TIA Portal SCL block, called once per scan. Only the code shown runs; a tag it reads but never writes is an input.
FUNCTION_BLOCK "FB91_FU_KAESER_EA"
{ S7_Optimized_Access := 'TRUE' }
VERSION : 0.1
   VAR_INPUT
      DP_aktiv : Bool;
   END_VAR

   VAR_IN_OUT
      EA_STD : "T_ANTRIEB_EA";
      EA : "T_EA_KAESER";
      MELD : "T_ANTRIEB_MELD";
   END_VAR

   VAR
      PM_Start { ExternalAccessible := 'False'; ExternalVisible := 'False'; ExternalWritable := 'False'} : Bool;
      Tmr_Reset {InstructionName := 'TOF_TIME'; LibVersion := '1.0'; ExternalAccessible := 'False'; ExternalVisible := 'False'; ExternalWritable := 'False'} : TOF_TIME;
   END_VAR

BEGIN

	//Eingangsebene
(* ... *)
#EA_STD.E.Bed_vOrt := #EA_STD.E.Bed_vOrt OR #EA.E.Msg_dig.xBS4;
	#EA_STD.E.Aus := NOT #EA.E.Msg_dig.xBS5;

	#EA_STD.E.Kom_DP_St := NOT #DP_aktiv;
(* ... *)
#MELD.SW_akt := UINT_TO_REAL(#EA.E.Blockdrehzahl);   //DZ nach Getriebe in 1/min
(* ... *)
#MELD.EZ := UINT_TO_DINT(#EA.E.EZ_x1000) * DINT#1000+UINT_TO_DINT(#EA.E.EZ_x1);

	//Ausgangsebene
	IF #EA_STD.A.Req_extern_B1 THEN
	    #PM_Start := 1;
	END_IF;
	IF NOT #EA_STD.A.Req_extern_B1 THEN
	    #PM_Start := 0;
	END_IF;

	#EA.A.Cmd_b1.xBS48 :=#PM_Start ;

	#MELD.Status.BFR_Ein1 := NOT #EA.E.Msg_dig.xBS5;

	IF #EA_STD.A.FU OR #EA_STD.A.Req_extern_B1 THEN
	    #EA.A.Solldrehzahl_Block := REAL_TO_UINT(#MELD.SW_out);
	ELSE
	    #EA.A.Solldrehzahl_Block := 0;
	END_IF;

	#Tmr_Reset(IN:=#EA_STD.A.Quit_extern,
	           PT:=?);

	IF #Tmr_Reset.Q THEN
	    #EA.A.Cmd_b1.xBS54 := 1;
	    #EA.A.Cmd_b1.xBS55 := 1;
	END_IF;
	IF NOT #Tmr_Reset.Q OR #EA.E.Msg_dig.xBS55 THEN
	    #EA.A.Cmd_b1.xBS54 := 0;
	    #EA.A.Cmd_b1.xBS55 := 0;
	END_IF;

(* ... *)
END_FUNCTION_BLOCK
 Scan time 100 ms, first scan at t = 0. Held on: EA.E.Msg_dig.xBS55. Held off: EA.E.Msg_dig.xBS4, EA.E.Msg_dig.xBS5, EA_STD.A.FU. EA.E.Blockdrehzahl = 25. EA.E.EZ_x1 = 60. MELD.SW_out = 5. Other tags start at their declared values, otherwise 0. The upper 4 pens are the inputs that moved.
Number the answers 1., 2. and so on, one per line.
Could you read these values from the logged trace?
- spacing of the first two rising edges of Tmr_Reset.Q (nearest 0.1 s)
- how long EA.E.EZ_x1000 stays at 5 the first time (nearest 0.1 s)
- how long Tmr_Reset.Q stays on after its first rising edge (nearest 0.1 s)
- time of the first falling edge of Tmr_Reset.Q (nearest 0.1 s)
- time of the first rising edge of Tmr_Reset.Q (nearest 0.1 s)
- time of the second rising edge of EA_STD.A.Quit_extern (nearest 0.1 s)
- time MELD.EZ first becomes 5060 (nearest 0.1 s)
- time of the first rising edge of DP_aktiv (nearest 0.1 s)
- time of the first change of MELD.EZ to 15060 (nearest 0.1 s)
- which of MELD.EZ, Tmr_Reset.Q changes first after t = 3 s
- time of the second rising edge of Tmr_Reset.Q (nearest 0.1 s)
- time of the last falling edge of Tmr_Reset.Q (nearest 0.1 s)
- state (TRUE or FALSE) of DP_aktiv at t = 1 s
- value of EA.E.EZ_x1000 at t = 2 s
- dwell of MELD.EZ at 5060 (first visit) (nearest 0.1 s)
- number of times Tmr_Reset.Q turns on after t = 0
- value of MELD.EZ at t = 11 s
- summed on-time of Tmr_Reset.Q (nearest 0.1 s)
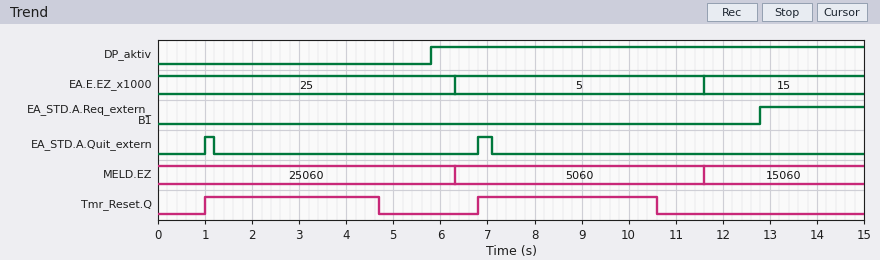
1. 5.8 s
2. 5.3 s
3. 3.7 s
4. 4.7 s
5. 1.0 s
6. 6.8 s
7. 6.3 s
8. 5.8 s
9. 11.6 s
10. Tmr_Reset.Q
11. 6.8 s
12. 10.6 s
13. FALSE
14. 25
15. 5.3 s
16. 2
17. 5060
18. 7.5 s
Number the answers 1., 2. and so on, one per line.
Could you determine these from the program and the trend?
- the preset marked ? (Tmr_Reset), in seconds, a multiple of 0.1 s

1. 3.5 s
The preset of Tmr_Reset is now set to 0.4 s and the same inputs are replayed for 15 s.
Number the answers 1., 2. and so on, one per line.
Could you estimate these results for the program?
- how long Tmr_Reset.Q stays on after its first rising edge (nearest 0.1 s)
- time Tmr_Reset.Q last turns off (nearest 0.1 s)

1. 0.6 s
2. 7.5 s
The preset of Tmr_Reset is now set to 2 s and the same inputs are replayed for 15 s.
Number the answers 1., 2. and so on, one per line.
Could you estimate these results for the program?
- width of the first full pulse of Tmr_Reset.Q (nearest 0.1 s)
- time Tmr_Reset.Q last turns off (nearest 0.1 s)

1. 2.2 s
2. 9.1 s
